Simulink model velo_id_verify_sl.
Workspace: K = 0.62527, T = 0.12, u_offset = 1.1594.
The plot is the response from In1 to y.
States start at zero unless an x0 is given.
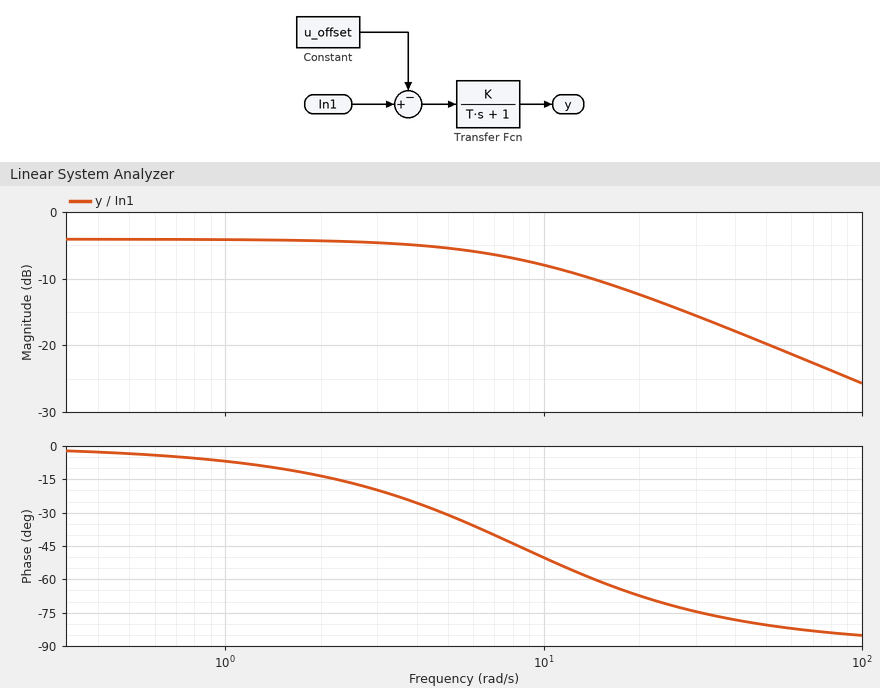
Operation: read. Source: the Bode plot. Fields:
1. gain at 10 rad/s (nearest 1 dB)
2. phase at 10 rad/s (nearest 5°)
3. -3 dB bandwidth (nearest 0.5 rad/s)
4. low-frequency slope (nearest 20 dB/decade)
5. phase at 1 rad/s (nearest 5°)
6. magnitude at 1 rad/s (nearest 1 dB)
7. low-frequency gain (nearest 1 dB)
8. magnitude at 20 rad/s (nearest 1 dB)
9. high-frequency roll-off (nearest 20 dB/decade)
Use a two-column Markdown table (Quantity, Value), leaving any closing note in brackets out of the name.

| Quantity | Value |
|---|---|
| gain at 10 rad/s | -8 dB |
| phase at 10 rad/s | -50° |
| -3 dB bandwidth | 8.5 rad/s |
| low-frequency slope | 0 dB/decade |
| phase at 1 rad/s | -5° |
| magnitude at 1 rad/s | -4 dB |
| low-frequency gain | -4 dB |
| magnitude at 20 rad/s | -12 dB |
| high-frequency roll-off | -20 dB/decade |
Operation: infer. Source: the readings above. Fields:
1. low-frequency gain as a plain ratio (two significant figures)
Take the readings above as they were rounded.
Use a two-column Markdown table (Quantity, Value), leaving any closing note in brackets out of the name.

| Quantity | Value |
|---|---|
| low-frequency gain as a plain ratio | 0.63 |
